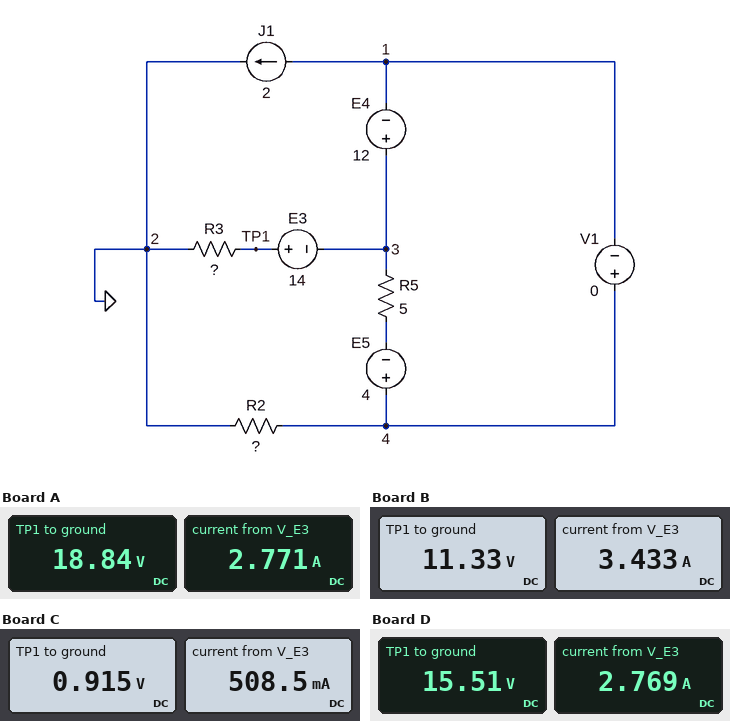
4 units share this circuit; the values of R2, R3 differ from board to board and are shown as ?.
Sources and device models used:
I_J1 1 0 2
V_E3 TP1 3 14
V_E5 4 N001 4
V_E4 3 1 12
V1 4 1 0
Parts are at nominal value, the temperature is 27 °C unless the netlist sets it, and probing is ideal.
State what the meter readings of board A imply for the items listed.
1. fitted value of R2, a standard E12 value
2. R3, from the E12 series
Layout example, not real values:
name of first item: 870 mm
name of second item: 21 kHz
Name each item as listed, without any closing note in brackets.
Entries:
fitted value of R2, a standard E12 value: 1.5 Ω
R3, from the E12 series: 6.8 Ω
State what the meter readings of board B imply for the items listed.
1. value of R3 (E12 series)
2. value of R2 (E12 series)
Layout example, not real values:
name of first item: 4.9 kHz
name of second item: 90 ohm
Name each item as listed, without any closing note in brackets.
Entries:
value of R3: 3.3 Ω
value of R2: 2.7 Ω
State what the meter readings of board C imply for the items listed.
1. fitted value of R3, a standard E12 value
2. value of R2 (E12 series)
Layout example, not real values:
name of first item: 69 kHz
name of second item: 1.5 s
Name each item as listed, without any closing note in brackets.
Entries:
fitted value of R3, a standard E12 value: 1.8 Ω
value of R2: 10 Ω
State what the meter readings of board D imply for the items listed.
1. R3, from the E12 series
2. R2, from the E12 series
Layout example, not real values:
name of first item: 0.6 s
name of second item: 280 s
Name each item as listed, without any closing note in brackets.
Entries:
R3, from the E12 series: 5.6 Ω
R2, from the E12 series: 2.2 Ω
